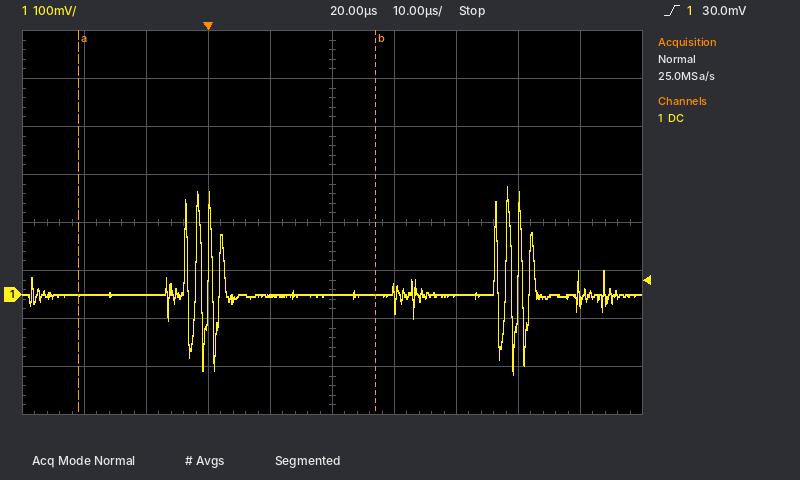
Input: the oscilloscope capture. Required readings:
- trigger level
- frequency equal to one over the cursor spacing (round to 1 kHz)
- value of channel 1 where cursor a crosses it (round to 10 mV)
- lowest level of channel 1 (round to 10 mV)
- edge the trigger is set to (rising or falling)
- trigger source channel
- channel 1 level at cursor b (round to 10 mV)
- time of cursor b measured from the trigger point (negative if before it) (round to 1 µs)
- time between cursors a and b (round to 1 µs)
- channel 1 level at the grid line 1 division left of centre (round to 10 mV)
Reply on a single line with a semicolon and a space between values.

30.0 mV; 21 kHz; 0 mV; -170 mV; rising; channel 1; 0 mV; +27 µs; 48 µs; 0 mV
